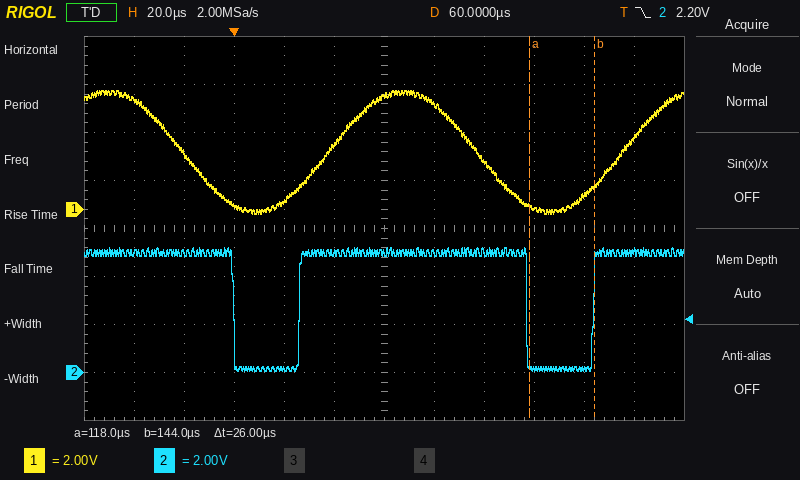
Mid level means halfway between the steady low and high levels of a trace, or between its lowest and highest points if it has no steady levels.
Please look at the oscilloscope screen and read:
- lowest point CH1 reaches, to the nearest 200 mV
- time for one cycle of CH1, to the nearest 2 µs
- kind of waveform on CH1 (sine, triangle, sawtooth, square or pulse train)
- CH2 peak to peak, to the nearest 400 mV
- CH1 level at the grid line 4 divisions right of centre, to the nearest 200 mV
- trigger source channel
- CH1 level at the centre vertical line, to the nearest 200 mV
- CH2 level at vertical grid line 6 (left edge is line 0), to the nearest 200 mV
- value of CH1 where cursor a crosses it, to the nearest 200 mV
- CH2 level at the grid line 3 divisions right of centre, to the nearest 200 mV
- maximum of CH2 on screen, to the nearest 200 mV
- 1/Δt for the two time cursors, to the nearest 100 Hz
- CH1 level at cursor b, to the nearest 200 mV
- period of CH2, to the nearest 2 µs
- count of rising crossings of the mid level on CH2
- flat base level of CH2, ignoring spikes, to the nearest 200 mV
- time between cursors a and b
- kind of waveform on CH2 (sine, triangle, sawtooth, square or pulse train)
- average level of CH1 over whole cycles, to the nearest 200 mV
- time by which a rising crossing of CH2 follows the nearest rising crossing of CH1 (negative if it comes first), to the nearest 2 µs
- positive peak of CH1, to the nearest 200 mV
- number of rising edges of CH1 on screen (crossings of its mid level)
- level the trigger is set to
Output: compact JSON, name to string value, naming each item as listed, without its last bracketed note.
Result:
{"lowest point CH1 reaches, to the nearest 200 mV": "-200 mV", "time for one cycle of CH1, to the nearest 2 µs": "118 µs", "kind of waveform on CH1": "sine", "CH2 peak to peak, to the nearest 400 mV": "5.2 V", "CH1 level at the grid line 4 divisions right of centre, to the nearest 200 mV": "600 mV", "trigger source channel": "CH2", "CH1 level at the centre vertical line, to the nearest 200 mV": "4.8 V", "CH2 level at vertical grid line 6 (left edge is line 0), to the nearest 200 mV": "5.0 V", "value of CH1 where cursor a crosses it, to the nearest 200 mV": "200 mV", "CH2 level at the grid line 3 divisions right of centre, to the nearest 200 mV": "200 mV", "maximum of CH2 on screen, to the nearest 200 mV": "5.2 V", "1/Δt for the two time cursors, to the nearest 100 Hz": "38.5 kHz", "CH1 level at cursor b, to the nearest 200 mV": "1.0 V", "period of CH2, to the nearest 2 µs": "118 µs", "count of rising crossings of the mid level on CH2": "2", "flat base level of CH2, ignoring spikes, to the nearest 200 mV": "200 mV", "time between cursors a and b": "26 µs", "kind of waveform on CH2": "pulse train", "average level of CH1 over whole cycles, to the nearest 200 mV": "2.4 V", "time by which a rising crossing of CH2 follows the nearest rising crossing of CH1 (negative if it comes first), to the nearest 2 µs": "-12 µs", "positive peak of CH1, to the nearest 200 mV": "5.0 V", "number of rising edges of CH1 on screen": "2", "level the trigger is set to": "2.20 V"}
